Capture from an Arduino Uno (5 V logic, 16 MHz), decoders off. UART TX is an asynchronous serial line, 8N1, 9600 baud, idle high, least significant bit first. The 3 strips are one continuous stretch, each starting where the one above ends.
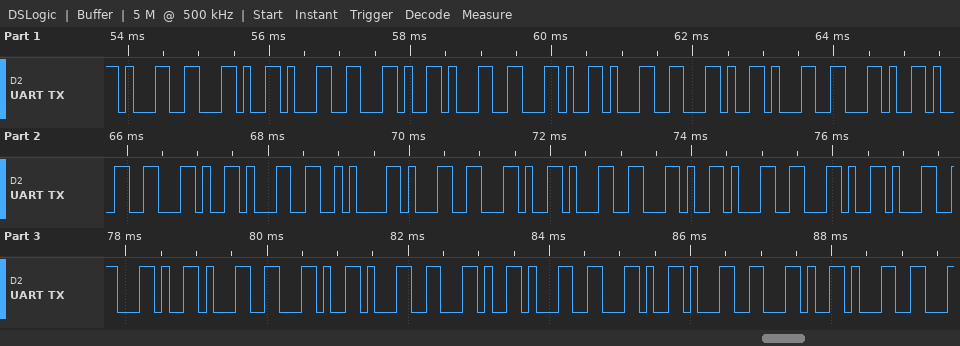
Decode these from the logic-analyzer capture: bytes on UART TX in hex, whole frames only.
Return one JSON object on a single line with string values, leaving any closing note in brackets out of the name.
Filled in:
{"bytes on UART TX in hex, whole frames only": "31 2C 31 2C 31 2C 31 2C 31 2C 31 2C 31 0A 31 2C 31 2C 31 2C 31 2C 31 2C 31 2C 31 2C 31 2C 31"}
